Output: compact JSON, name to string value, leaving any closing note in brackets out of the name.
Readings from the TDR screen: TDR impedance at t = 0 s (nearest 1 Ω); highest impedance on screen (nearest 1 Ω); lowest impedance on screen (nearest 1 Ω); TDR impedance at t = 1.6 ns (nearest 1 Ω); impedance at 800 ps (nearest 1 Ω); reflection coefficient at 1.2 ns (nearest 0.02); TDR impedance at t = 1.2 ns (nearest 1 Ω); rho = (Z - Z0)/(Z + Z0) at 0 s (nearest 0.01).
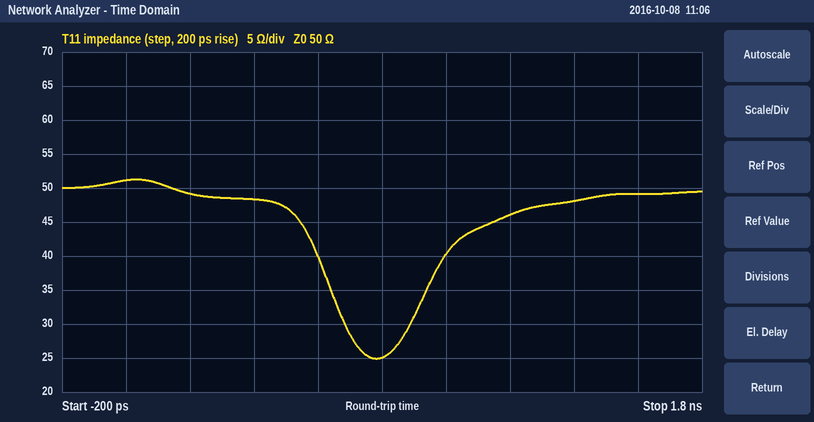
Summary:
{"TDR impedance at t = 0 s": "51 Ω", "highest impedance on screen": "51 Ω", "lowest impedance on screen": "25 Ω", "TDR impedance at t = 1.6 ns": "49 Ω", "impedance at 800 ps": "25 Ω", "reflection coefficient at 1.2 ns": "-0.04", "TDR impedance at t = 1.2 ns": "46 Ω", "rho = (Z - Z0)/(Z + Z0) at 0 s": "+0.01"}
